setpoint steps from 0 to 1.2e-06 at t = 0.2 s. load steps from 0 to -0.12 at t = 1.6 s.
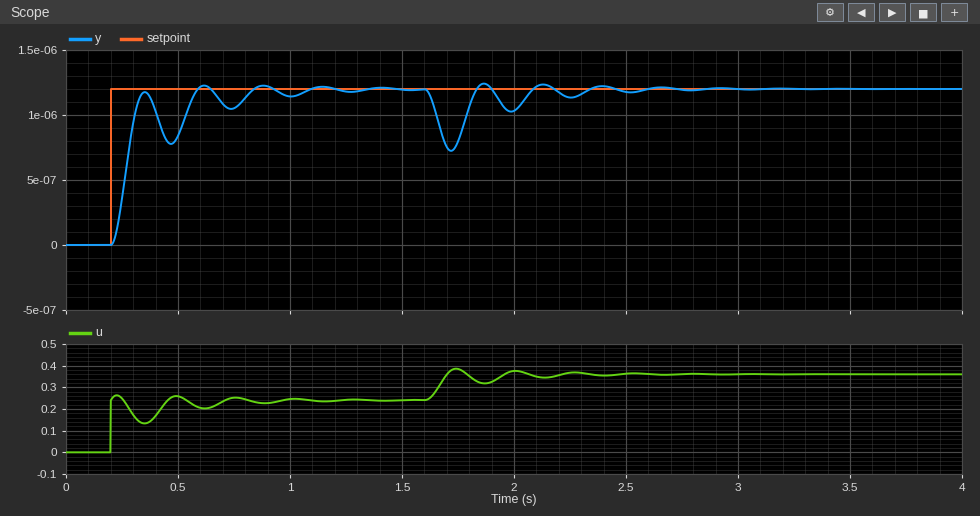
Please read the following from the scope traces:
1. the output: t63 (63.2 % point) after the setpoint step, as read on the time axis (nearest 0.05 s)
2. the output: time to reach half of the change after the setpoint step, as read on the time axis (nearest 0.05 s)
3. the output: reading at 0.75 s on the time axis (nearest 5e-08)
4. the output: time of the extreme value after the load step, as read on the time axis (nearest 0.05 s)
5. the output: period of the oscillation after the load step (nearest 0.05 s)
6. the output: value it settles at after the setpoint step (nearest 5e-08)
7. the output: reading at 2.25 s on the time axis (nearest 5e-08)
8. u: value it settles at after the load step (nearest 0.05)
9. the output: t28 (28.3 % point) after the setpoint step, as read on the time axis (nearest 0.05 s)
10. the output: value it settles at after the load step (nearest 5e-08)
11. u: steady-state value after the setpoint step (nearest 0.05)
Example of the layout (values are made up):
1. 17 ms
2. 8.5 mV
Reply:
1. 0.30 s
2. 0.25 s
3. 0.00000105
4. 1.70 s
5. 0.25 s
6. 0.00000120
7. 0.00000115
8. 0.35
9. 0.25 s
10. 0.00000120
11. 0.25
